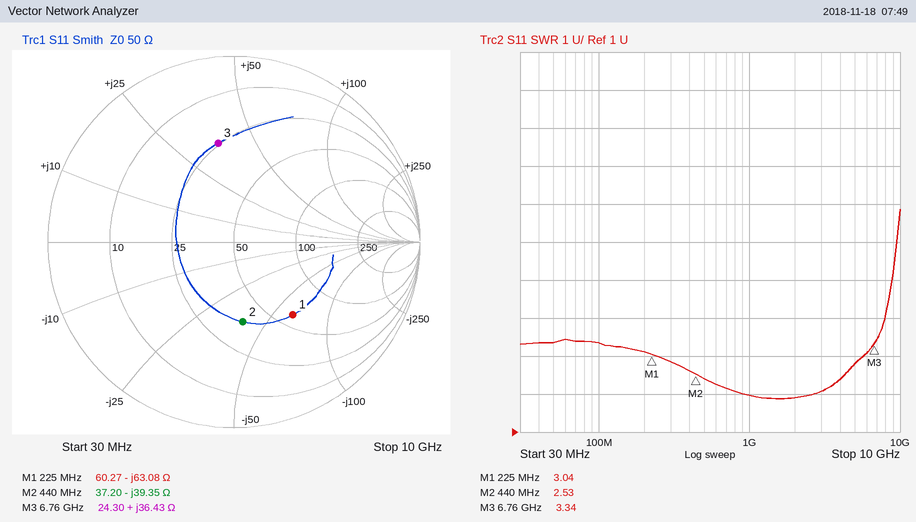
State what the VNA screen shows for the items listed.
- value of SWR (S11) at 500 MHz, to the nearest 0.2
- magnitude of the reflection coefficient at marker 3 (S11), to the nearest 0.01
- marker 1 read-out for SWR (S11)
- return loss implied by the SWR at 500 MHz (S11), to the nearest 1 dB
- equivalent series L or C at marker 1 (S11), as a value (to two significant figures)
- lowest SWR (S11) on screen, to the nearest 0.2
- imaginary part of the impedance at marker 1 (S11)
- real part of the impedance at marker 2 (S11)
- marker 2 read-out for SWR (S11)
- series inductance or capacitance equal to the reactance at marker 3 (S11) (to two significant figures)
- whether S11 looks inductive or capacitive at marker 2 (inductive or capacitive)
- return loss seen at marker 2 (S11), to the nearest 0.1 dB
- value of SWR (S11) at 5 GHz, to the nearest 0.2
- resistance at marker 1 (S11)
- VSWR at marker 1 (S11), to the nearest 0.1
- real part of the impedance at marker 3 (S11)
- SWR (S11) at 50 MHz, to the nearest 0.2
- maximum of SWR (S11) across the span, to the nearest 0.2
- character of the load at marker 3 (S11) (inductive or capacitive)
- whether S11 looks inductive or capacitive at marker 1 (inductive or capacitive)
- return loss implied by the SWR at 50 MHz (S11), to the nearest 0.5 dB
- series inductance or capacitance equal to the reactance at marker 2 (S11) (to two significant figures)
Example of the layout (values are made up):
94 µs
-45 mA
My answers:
2.4
0.54
3.04
8 dB
11 pF
1.8
-63.08 Ω
37.20 Ω
2.53
860 pH
capacitive
7.3 dB
2.8
60.27 Ω
3.0
24.30 Ω
3.4
6.8
inductive
capacitive
5.5 dB
9.2 pF
